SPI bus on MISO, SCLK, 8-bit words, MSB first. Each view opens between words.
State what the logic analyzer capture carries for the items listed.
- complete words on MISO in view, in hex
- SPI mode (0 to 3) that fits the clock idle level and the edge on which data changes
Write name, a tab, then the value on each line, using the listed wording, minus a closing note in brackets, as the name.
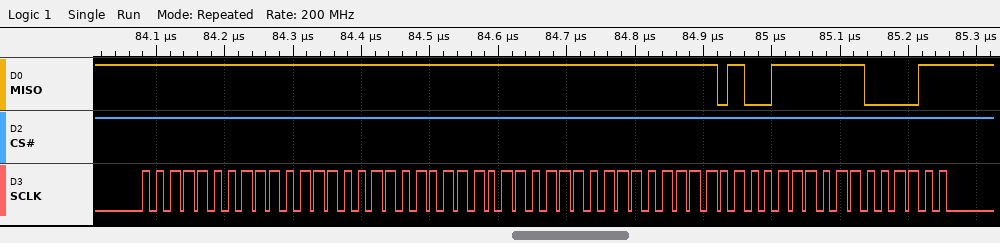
complete words on MISO in view, in hex	FF, FF, FF, FF, FF, 4F, C3
SPI mode (0 to 3) that fits the clock idle level and the edge on which data changes	0
